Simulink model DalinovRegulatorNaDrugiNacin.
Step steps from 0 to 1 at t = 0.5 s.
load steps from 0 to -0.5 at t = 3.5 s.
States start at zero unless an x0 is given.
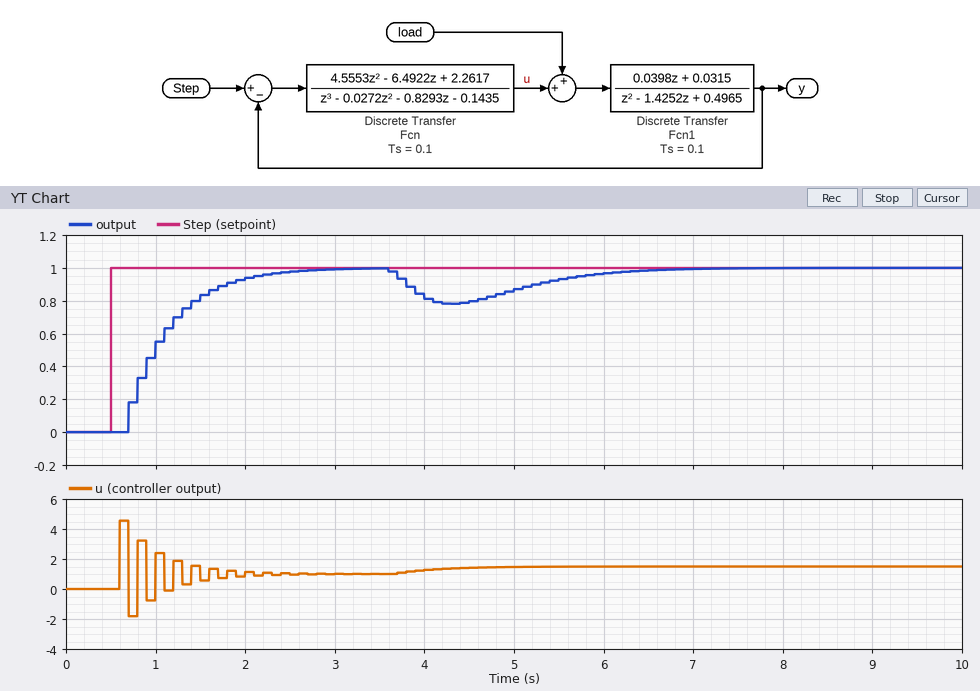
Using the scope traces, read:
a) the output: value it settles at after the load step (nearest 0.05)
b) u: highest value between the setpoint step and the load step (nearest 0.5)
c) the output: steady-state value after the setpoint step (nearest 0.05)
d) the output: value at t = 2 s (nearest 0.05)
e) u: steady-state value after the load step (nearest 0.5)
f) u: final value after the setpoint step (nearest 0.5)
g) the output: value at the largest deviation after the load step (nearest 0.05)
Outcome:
1.00
4.5
1.00
0.95
1.5
1.0
0.80
